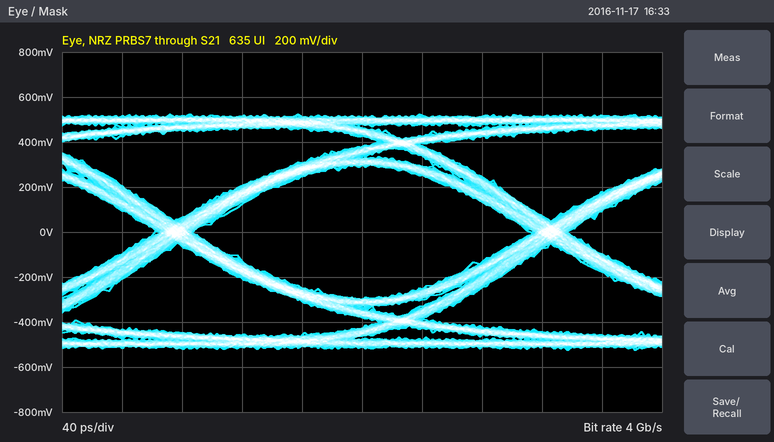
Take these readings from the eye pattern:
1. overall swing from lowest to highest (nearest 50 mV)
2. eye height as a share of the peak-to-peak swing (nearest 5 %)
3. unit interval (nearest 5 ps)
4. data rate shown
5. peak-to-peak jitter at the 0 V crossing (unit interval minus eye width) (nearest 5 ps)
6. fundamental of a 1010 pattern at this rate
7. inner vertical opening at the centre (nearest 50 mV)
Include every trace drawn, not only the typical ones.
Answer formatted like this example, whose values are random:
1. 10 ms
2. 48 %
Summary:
1. 1.05 V
2. 55 %
3. 250 ps
4. 4 Gb/s
5. 25 ps
6. 2 GHz
7. 600 mV
